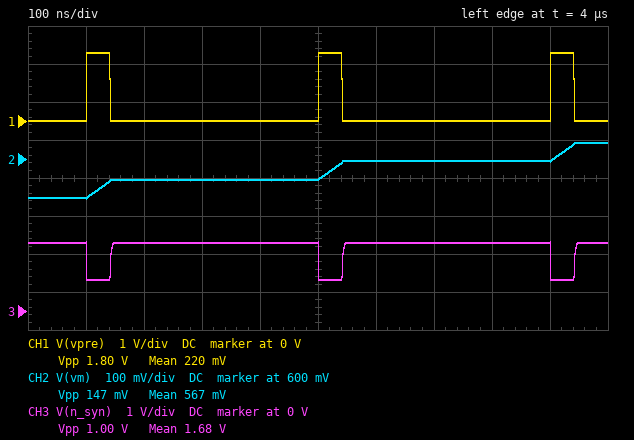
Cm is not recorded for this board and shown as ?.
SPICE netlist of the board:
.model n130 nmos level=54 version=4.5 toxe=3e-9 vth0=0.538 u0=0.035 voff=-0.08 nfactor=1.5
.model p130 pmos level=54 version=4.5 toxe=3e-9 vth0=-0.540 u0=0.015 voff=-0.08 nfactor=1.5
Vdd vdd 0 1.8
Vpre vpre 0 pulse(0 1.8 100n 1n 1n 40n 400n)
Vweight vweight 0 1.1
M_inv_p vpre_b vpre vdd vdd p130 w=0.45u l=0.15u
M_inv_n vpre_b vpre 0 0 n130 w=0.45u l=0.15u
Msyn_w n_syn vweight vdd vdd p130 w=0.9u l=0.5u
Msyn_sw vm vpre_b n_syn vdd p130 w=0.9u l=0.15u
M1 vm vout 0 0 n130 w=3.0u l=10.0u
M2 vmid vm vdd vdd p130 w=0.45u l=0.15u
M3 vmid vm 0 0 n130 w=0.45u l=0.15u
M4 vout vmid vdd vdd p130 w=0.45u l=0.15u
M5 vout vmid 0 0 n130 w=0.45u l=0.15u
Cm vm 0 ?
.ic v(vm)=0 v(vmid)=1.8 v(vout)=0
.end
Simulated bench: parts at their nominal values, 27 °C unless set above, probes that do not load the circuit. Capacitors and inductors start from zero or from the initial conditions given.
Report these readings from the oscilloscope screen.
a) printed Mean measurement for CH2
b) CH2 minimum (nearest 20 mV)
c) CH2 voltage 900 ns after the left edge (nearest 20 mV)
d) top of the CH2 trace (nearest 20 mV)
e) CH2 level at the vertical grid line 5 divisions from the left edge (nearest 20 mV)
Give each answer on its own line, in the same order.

567 mV
500 mV
600 mV
640 mV
540 mV
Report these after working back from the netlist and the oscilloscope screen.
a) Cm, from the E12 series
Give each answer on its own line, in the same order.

390 fF
